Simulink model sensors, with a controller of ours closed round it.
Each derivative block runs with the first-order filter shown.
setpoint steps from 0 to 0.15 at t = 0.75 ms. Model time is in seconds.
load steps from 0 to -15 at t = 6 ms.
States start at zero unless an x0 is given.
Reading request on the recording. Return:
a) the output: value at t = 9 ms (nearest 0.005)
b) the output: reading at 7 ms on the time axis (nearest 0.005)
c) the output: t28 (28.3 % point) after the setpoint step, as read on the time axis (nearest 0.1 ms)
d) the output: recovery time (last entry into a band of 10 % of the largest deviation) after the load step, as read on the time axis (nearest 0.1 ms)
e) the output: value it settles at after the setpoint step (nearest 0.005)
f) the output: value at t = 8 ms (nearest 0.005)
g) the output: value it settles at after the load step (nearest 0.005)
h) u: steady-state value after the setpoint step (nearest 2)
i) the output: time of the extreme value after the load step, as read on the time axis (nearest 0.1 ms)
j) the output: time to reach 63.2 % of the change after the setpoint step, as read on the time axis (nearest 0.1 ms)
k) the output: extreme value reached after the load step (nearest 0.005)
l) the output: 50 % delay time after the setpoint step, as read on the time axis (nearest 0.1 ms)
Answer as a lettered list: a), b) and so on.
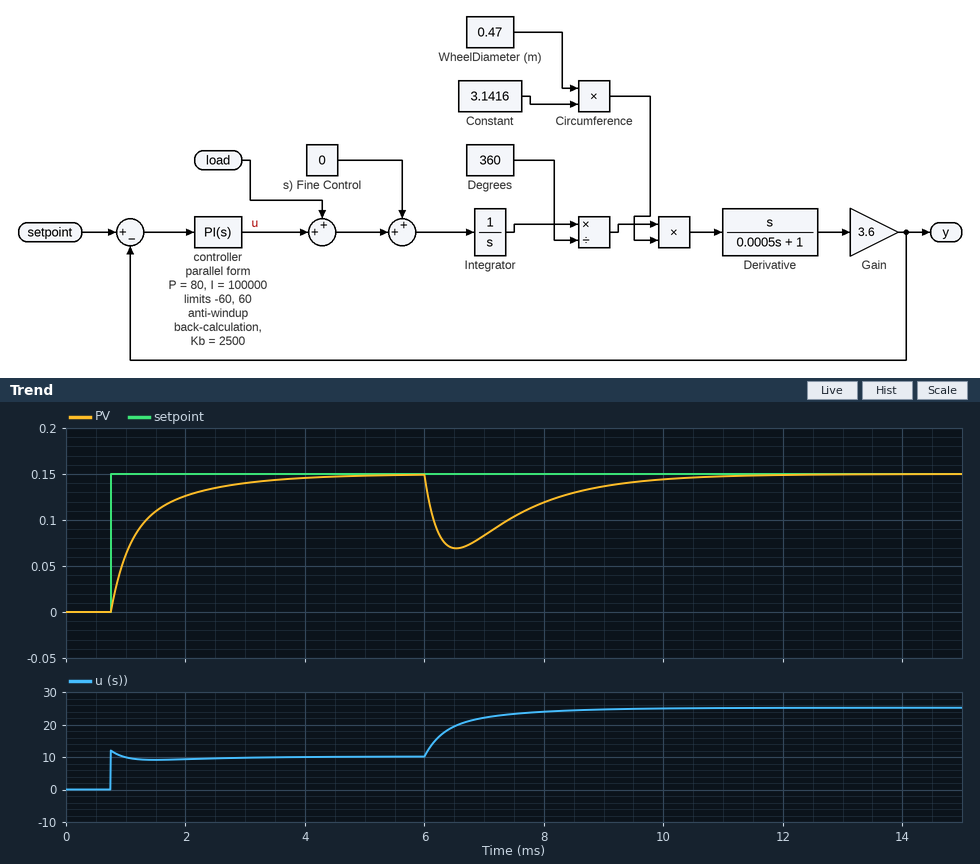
a) 0.135
b) 0.085
c) 0.9 ms
d) 9.6 ms
e) 0.150
f) 0.120
g) 0.150
h) 10
i) 6.5 ms
j) 1.3 ms
k) 0.070
l) 1.1 ms
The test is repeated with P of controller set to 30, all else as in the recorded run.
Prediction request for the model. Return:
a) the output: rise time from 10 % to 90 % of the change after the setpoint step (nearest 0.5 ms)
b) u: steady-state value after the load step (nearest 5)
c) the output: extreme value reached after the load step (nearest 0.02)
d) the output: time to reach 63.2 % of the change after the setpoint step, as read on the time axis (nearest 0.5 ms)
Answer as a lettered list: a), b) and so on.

a) 1.5 ms
b) 25
c) 0.04
d) 1.5 ms
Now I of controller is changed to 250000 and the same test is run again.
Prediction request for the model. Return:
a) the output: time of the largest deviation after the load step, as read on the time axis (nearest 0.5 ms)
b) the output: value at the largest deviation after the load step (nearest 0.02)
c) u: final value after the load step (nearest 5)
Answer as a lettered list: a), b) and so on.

a) 6.5 ms
b) 0.08
c) 25
